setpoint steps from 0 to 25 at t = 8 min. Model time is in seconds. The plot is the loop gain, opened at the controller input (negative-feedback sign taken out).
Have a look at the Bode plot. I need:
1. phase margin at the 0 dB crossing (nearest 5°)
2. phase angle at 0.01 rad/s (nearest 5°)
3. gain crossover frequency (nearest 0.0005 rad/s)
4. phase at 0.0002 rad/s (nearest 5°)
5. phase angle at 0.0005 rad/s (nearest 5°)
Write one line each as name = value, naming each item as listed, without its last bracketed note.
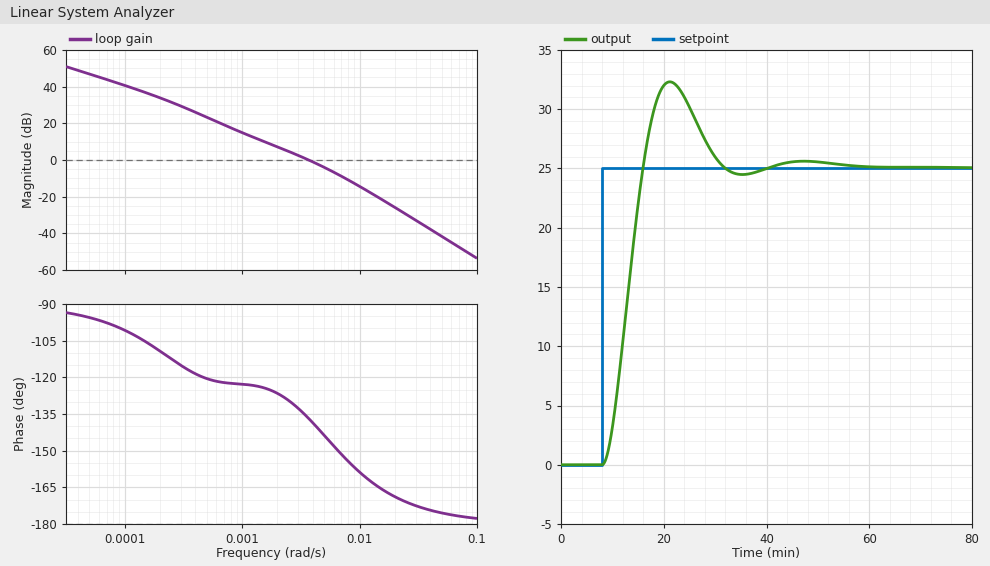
phase margin at the 0 dB crossing = 45°
phase angle at 0.01 rad/s = -160°
gain crossover frequency = 0.0035 rad/s
phase at 0.0002 rad/s = -110°
phase angle at 0.0005 rad/s = -120°
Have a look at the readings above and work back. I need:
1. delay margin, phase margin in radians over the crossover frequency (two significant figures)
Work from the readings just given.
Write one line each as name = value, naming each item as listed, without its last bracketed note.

delay margin, phase margin in radians over the crossover frequency = 220 s
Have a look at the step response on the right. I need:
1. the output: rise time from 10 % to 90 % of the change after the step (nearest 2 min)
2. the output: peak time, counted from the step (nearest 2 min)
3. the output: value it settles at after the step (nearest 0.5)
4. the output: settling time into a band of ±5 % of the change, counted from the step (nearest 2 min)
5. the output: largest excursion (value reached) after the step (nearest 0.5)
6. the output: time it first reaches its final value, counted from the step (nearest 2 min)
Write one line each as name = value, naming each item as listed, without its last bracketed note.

the output: rise time from 10 % to 90 % of the change after the step = 6 min
the output: peak time, counted from the step = 14 min
the output: value it settles at after the step = 25.0
the output: settling time into a band of ±5 % of the change, counted from the step = 22 min
the output: largest excursion (value reached) after the step = 32.5
the output: time it first reaches its final value, counted from the step = 8 min
